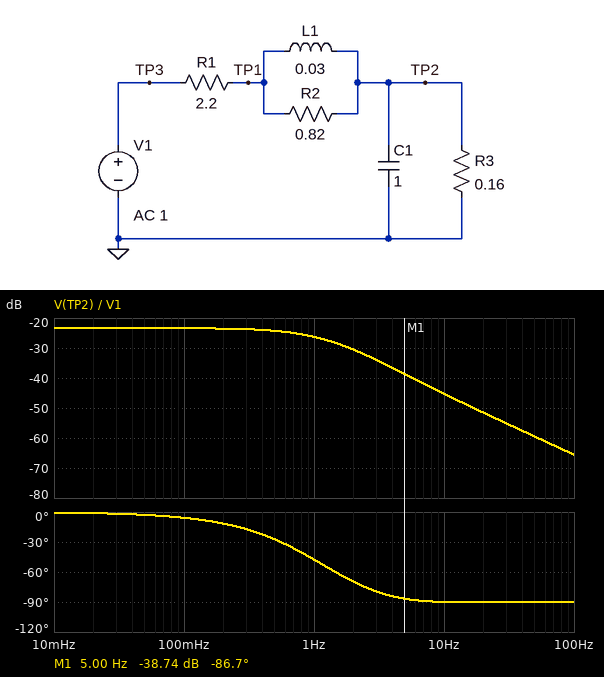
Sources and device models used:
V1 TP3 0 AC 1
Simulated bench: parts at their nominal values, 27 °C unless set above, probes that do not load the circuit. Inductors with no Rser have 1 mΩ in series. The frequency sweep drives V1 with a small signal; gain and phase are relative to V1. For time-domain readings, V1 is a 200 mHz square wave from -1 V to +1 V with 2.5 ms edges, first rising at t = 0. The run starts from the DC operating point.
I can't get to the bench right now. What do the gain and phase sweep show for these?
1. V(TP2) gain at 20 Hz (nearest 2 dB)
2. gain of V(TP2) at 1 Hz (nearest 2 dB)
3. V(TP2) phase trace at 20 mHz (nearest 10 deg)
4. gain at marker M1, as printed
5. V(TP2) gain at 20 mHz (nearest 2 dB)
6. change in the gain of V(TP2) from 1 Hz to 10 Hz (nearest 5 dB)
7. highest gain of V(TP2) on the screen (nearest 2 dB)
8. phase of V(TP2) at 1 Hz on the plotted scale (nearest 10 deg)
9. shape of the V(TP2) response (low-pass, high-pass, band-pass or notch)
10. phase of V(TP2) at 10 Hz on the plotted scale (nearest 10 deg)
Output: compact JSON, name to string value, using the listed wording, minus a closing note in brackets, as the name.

{"V(TP2) gain at 20 Hz": "-52 dB", "gain of V(TP2) at 1 Hz": "-26 dB", "V(TP2) phase trace at 20 mHz": "0 deg", "gain at marker M1, as printed": "-38.74 dB", "V(TP2) gain at 20 mHz": "-24 dB", "change in the gain of V(TP2) from 1 Hz to 10 Hz": "-20 dB", "highest gain of V(TP2) on the screen": "-24 dB", "phase of V(TP2) at 1 Hz on the plotted scale": "-50 deg", "shape of the V(TP2) response": "low-pass", "phase of V(TP2) at 10 Hz on the plotted scale": "-90 deg"}
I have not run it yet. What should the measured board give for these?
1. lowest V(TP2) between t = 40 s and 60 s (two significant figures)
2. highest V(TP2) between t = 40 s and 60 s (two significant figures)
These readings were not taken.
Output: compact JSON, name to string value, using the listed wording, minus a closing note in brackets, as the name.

{"lowest V(TP2) between t = 40 s and 60 s": "-68 mV", "highest V(TP2) between t = 40 s and 60 s": "68 mV"}
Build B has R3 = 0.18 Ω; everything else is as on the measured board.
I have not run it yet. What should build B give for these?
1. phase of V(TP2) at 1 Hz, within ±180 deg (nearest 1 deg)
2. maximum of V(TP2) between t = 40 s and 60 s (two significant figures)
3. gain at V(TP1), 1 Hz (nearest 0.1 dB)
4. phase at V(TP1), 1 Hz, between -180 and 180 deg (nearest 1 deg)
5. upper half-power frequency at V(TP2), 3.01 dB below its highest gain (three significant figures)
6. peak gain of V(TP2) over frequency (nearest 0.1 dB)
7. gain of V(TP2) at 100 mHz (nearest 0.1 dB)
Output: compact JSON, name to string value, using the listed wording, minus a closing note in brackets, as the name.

{"phase of V(TP2) at 1 Hz, within ±180 deg": "-51 deg", "maximum of V(TP2) between t = 40 s and 60 s": "76 mV", "gain at V(TP1), 1 Hz": "-23.8 dB", "phase at V(TP1), 1 Hz, between -180 and 180 deg": "34 deg", "upper half-power frequency at V(TP2), 3.01 dB below its highest gain": "927 mHz", "peak gain of V(TP2) over frequency": "-22.4 dB", "gain of V(TP2) at 100 mHz": "-22.5 dB"}
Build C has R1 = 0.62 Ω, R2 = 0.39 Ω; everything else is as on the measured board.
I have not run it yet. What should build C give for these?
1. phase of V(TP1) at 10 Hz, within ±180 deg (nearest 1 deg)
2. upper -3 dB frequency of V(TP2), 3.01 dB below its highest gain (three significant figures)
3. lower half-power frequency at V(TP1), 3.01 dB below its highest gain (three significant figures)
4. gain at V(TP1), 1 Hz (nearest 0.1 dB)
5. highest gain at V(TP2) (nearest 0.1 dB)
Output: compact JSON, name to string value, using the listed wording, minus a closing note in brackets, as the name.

{"phase of V(TP1) at 10 Hz, within ±180 deg": "6 deg", "upper -3 dB frequency of V(TP2), 3.01 dB below its highest gain": "1.00 Hz", "lower half-power frequency at V(TP1), 3.01 dB below its highest gain": "1.60 Hz", "gain at V(TP1), 1 Hz": "-13.2 dB", "highest gain at V(TP2)": "-13.8 dB"}
